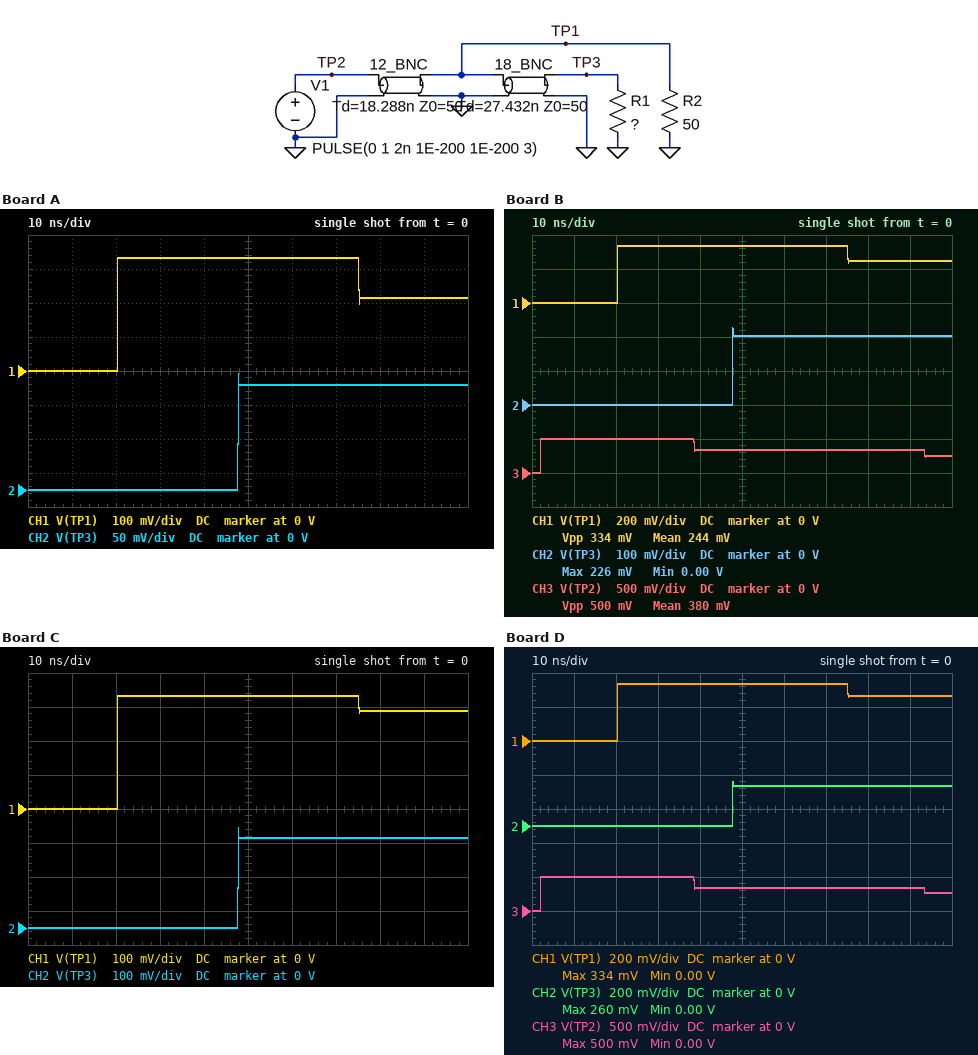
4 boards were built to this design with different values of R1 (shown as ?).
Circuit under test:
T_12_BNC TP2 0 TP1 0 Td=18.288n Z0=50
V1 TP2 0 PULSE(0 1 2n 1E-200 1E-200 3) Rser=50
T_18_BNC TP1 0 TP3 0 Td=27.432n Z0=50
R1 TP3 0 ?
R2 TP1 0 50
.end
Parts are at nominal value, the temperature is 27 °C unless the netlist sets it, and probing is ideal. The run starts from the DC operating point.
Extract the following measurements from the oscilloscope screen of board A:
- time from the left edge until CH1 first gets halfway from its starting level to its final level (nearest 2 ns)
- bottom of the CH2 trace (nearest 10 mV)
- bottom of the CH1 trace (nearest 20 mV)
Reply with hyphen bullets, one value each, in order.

- 20 ns
- 0 V
- 0 V
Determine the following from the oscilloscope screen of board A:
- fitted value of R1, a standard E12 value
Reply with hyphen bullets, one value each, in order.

- 15 Ω
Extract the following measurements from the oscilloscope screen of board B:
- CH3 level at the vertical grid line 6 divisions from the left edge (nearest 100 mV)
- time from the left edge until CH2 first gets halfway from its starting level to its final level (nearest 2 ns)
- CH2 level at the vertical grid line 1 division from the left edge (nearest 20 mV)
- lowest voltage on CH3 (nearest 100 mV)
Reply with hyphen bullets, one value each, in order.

- 300 mV
- 48 ns
- 0 V
- 0 V
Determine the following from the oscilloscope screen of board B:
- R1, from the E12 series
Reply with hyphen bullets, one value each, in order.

- 22 Ω
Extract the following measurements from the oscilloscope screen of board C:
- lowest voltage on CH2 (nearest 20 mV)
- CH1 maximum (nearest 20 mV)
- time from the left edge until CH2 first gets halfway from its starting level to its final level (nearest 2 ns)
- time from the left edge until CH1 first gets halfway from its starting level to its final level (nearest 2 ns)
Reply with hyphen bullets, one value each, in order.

- 0 V
- 340 mV
- 48 ns
- 20 ns
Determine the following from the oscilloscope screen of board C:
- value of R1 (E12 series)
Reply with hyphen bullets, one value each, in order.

- 33 Ω
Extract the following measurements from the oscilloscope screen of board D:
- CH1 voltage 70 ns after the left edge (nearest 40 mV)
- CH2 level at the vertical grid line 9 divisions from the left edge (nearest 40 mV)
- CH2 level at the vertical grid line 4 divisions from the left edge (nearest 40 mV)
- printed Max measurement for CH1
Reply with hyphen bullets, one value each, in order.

- 320 mV
- 240 mV
- 0 V
- 334 mV
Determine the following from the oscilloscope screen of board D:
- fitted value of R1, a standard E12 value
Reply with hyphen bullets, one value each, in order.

- 27 Ω
